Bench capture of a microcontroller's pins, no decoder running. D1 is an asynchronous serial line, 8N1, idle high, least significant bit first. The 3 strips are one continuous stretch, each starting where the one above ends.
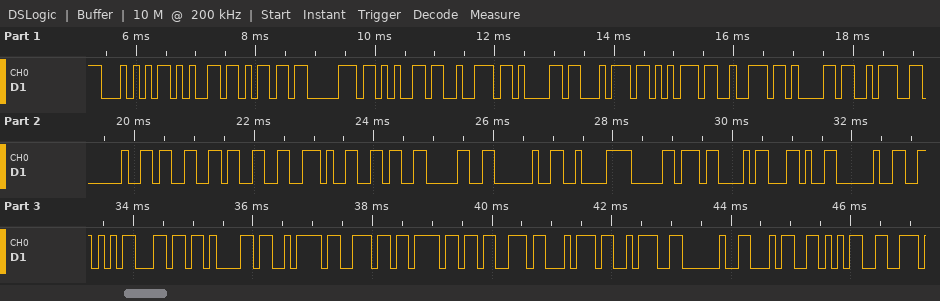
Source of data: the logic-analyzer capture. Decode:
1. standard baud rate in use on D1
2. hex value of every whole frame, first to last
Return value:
9600 baud
54 65 6D 70 65 72 61 74 75 72 61 3A 20 33 33 2E 36 30 20 C2 B0 43 2C 20 56 6C 61 7A 6E 6F 73 74 3A 20 34 35
